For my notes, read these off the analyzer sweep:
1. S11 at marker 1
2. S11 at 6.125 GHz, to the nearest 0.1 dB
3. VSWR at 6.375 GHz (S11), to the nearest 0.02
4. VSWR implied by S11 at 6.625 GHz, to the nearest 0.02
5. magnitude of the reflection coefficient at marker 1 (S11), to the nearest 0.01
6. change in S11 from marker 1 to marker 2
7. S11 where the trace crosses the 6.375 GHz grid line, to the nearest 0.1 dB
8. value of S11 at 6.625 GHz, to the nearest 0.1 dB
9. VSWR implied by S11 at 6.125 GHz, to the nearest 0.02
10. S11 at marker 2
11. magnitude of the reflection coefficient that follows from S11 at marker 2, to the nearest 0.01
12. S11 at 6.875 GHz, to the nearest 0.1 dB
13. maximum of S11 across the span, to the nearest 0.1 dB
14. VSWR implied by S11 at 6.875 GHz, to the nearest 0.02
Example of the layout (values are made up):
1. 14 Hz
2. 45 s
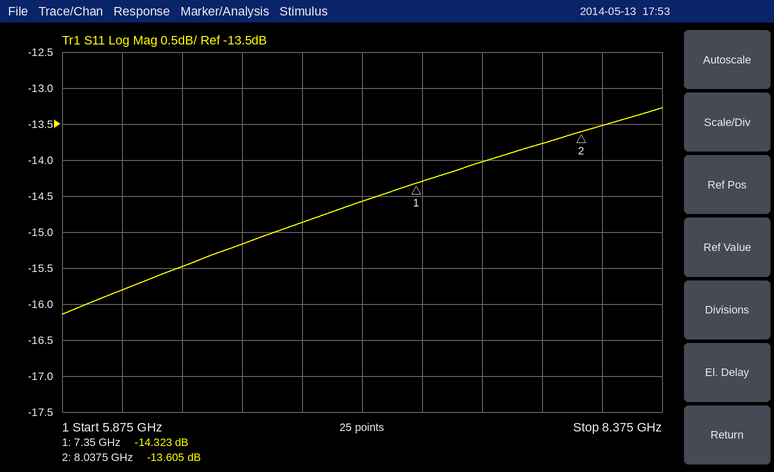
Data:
1. -14.323 dB
2. -15.8 dB
3. 1.40
4. 1.42
5. 0.19
6. 0.718 dB
7. -15.5 dB
8. -15.2 dB
9. 1.38
10. -13.605 dB
11. 0.21
12. -14.9 dB
13. -13.3 dB
14. 1.44
